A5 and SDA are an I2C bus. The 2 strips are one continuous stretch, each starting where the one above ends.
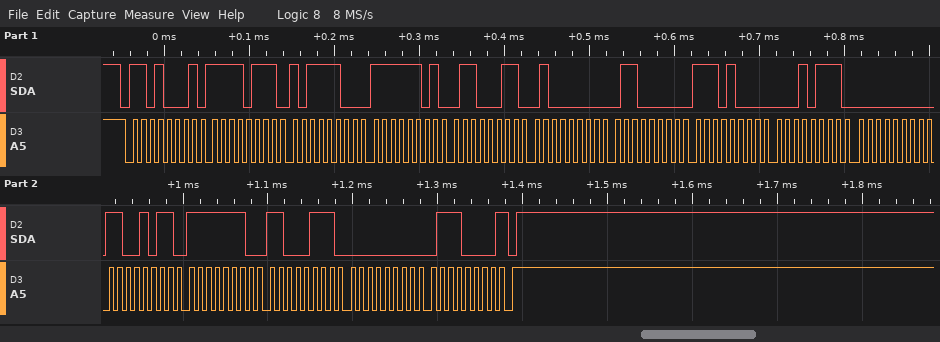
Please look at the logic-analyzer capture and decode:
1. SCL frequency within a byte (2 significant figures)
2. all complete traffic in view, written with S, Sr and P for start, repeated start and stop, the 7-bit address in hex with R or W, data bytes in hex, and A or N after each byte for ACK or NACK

100 kHz
S 68R A F7 A BC A FD A 63 A 40 A 60 A E8 A 17 A 00 A CB A FE A C7 A 00 A 70 N P
